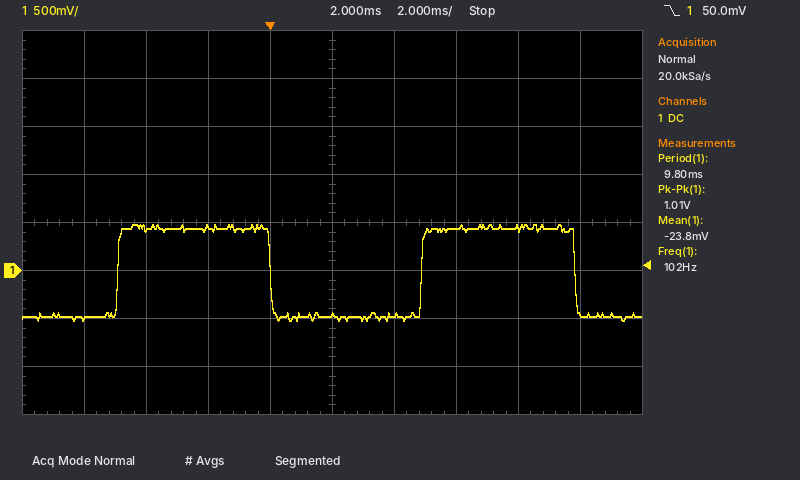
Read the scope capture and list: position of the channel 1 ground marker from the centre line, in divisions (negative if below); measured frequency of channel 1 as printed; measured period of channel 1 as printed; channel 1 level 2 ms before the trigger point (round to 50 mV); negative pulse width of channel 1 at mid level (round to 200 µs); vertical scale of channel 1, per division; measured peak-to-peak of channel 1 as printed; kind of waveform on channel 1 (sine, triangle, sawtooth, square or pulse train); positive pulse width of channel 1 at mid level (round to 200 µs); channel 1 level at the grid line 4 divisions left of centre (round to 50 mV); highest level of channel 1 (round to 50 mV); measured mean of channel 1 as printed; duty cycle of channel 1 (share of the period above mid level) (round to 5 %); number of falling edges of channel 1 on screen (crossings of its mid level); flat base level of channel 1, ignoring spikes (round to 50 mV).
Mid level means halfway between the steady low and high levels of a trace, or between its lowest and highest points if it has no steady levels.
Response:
-1.0 div
102 Hz
9.80 ms
450 mV
4.8 ms
500 mV
1.01 V
square
5.0 ms
-500 mV
500 mV
-23.8 mV
50 %
2
-500 mV
